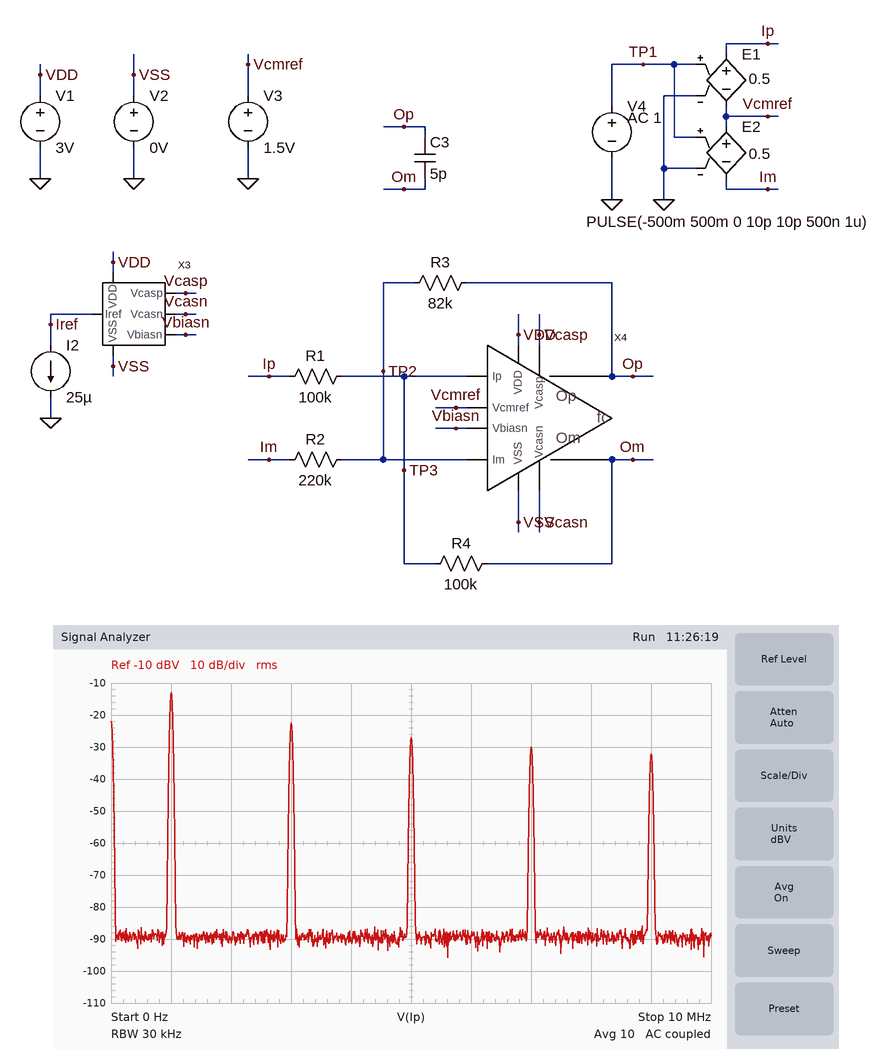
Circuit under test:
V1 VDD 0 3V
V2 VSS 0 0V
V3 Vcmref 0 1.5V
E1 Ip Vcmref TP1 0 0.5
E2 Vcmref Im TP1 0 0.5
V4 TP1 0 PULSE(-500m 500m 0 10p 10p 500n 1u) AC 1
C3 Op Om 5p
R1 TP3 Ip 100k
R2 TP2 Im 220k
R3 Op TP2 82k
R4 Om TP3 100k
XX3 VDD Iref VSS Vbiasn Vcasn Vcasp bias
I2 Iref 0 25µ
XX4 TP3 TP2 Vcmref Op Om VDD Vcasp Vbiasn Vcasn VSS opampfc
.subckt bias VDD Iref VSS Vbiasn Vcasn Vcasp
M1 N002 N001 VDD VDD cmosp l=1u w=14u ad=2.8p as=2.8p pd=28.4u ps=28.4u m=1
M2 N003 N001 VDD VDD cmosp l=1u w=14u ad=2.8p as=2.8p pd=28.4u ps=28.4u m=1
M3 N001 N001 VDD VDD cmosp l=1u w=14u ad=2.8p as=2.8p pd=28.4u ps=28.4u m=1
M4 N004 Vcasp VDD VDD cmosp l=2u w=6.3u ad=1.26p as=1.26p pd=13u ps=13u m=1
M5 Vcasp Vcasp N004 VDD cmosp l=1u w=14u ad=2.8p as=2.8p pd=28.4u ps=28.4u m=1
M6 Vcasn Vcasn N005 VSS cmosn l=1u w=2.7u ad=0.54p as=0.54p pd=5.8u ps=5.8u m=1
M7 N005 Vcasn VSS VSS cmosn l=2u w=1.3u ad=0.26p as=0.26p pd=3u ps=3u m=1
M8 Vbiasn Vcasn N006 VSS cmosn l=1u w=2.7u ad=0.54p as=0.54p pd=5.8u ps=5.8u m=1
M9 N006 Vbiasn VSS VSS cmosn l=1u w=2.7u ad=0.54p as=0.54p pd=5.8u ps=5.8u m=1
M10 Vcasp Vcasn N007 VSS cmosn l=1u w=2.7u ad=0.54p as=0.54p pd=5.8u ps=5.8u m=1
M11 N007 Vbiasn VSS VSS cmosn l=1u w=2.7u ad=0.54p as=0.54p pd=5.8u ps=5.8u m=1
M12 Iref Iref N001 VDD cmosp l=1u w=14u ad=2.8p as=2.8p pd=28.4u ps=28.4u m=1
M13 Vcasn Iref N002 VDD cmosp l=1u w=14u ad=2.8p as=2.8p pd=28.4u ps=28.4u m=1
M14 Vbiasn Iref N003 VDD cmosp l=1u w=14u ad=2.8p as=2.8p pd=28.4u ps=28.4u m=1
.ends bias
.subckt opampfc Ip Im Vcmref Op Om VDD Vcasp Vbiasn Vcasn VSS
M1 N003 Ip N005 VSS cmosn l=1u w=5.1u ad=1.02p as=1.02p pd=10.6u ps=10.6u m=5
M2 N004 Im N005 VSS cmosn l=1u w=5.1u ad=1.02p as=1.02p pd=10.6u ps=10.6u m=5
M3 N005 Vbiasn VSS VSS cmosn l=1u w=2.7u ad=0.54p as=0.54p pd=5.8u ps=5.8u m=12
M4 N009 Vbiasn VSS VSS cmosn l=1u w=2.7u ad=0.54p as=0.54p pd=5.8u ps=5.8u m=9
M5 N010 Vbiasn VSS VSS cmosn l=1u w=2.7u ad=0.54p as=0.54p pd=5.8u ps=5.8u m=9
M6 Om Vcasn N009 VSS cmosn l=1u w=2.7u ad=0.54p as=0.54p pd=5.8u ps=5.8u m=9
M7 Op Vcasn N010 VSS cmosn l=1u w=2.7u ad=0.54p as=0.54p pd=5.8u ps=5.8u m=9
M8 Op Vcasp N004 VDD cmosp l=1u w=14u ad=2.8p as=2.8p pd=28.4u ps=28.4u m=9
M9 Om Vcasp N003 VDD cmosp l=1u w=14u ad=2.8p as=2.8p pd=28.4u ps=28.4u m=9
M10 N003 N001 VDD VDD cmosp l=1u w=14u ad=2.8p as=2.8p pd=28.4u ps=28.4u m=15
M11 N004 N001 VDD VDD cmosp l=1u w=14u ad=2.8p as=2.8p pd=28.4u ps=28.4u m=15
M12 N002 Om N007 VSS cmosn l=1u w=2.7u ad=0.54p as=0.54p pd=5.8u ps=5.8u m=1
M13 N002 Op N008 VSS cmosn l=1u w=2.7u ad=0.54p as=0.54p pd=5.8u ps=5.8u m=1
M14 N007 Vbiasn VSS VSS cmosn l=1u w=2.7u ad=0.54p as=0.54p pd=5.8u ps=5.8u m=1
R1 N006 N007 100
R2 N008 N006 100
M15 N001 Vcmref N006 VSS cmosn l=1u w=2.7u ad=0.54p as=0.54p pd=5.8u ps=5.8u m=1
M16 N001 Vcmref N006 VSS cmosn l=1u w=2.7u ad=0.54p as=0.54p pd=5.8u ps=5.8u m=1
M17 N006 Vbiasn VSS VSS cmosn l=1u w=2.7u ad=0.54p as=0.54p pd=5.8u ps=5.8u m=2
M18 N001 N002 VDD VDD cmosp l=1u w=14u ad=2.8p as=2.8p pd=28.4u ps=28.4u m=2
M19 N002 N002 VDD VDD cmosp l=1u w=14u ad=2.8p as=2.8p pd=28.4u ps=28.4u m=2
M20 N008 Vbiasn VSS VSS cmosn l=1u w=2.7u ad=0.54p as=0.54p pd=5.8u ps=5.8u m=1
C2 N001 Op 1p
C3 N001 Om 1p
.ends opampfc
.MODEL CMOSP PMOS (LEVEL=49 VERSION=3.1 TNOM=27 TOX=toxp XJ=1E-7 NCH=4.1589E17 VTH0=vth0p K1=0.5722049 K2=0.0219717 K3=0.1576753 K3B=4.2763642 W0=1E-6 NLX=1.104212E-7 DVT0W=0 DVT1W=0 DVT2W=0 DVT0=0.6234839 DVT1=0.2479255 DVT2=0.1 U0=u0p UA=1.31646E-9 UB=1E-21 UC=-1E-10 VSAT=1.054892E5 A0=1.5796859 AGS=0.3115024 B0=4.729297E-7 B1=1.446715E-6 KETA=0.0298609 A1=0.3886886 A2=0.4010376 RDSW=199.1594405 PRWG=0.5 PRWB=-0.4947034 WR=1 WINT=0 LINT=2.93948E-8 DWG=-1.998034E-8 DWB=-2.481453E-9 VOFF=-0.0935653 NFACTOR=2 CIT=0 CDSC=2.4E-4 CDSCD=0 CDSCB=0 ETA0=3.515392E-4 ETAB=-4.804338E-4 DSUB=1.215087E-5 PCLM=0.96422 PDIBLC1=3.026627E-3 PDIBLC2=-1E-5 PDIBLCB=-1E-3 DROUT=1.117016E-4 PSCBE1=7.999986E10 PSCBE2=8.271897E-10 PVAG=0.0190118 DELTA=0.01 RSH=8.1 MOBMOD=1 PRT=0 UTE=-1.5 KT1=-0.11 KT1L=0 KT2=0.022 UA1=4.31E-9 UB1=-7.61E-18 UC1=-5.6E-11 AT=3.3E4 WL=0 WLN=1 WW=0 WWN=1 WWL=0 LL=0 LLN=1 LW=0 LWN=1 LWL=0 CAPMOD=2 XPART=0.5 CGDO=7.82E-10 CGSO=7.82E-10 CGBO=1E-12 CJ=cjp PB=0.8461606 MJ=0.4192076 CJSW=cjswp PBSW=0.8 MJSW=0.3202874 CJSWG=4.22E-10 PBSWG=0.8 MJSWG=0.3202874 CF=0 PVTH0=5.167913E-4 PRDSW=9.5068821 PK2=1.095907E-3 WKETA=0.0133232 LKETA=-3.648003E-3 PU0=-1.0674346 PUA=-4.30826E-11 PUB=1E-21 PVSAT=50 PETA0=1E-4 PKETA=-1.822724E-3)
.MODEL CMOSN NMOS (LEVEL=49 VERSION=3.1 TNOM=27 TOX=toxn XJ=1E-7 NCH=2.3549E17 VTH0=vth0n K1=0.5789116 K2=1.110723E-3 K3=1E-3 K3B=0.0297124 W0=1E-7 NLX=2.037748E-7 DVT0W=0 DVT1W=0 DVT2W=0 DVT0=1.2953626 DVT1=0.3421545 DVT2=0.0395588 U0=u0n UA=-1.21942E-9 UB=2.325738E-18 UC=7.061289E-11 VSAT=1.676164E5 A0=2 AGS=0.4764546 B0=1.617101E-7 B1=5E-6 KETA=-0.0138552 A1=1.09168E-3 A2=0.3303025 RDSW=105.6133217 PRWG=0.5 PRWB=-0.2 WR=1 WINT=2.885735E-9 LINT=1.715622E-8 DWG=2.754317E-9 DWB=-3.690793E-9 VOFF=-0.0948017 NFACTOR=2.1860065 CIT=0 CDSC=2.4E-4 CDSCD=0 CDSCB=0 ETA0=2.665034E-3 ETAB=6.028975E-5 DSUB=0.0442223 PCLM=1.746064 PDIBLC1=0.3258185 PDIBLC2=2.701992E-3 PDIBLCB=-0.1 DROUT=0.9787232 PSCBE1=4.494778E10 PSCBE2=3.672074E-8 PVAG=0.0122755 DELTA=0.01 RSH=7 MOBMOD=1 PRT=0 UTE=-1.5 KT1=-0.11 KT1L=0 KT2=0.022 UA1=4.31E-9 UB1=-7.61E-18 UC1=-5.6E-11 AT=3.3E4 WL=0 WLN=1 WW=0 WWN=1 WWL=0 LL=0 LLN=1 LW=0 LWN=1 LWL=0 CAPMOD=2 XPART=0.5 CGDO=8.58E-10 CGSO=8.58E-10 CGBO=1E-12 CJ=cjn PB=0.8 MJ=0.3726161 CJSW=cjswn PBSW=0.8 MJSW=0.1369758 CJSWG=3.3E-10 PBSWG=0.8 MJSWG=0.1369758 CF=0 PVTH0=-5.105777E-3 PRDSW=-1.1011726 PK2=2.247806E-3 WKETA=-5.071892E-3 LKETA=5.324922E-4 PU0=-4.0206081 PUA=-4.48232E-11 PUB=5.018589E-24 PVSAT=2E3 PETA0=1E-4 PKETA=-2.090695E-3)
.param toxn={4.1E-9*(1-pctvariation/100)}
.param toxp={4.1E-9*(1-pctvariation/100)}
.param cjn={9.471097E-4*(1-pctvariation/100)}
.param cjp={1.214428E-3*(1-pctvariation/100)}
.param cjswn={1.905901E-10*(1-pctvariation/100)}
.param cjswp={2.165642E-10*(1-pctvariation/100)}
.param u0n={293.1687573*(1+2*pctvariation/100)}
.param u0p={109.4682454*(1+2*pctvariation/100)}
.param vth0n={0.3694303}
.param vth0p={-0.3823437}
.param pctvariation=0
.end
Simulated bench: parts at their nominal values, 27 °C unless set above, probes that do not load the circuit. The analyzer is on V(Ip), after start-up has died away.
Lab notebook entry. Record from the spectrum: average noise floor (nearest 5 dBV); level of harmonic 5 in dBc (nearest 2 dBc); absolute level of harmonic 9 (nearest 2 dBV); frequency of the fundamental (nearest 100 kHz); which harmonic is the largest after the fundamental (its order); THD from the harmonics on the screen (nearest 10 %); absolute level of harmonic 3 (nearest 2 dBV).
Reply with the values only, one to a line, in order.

-90 dBV
-14 dBc
-32 dBV
1.0 MHz
3
40 %
-22 dBV
